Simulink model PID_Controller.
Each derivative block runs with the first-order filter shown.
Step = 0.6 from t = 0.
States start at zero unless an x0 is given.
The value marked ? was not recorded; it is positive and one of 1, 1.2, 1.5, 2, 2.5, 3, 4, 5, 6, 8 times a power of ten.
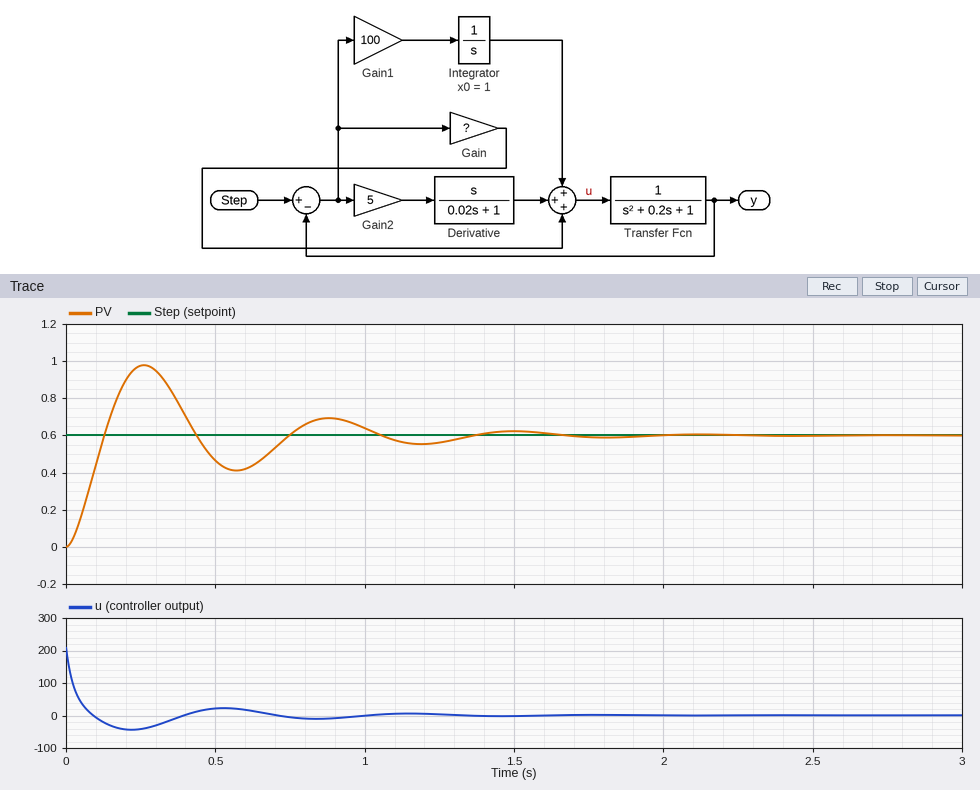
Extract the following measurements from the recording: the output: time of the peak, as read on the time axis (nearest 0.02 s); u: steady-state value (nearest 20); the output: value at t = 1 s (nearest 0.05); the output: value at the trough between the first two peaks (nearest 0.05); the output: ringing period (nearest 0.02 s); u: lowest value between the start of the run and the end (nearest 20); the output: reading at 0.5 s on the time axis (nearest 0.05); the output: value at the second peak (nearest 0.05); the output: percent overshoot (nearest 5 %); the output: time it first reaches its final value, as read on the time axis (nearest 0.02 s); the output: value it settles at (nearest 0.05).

0.26 s
0
0.65
0.40
0.62 s
-40
0.45
0.70
65 %
0.12 s
0.60
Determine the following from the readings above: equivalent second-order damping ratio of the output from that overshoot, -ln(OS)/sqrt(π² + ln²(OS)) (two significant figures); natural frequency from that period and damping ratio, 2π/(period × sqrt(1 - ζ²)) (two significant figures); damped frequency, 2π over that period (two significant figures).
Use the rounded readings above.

0.14
10 rad/s
10 rad/s
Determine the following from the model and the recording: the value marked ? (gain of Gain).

100
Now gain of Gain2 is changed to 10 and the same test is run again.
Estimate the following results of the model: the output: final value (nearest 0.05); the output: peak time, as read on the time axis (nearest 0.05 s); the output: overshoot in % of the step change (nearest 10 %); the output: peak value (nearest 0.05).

0.60
0.20 s
40 %
0.85
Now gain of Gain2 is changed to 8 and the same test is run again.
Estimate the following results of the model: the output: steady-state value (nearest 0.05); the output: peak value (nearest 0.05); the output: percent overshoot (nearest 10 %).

0.60
0.90
50 %
